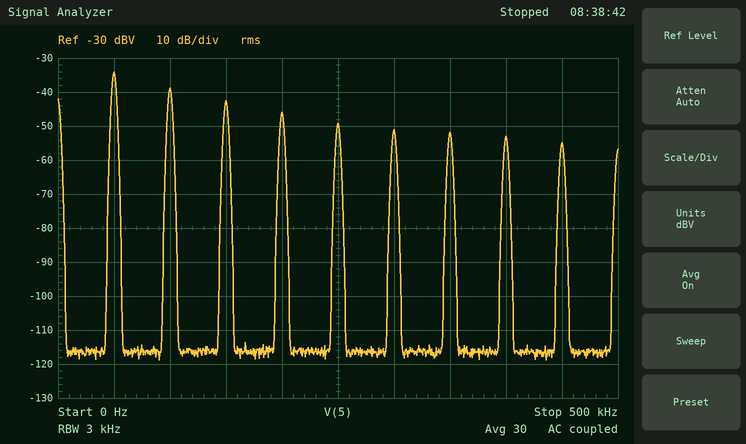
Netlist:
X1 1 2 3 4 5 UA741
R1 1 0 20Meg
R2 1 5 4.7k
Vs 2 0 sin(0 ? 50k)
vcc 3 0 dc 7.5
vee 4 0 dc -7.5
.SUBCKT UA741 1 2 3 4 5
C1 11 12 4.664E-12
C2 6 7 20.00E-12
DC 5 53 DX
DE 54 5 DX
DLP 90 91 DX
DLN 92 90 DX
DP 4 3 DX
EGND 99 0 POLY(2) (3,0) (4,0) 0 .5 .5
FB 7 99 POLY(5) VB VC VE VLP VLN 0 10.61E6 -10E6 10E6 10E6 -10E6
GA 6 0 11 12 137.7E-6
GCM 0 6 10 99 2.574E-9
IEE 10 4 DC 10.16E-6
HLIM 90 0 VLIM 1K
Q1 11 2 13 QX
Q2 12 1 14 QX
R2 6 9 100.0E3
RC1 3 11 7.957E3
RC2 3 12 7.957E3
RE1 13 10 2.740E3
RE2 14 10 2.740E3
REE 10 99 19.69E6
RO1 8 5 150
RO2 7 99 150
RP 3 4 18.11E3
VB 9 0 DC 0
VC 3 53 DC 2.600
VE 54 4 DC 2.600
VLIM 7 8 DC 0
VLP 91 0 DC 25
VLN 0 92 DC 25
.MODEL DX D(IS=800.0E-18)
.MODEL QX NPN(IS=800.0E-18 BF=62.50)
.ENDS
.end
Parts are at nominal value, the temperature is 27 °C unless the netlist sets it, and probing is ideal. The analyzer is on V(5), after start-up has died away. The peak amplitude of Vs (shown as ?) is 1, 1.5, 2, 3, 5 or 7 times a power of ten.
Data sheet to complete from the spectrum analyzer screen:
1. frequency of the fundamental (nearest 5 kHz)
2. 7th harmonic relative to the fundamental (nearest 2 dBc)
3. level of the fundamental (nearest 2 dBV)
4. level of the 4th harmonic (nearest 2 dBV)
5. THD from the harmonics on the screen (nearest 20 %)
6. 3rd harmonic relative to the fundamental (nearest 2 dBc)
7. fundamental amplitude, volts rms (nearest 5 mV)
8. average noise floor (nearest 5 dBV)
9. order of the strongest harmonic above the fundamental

50 kHz
-18 dBc
-34 dBV
-46 dBV
80 %
-8 dBc
20 mV
-115 dBV
2
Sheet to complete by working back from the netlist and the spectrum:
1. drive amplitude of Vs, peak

10 V
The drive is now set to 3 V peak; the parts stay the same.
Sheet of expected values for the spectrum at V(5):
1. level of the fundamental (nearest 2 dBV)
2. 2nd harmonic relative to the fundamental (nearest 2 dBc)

-72 dBV
-50 dBc
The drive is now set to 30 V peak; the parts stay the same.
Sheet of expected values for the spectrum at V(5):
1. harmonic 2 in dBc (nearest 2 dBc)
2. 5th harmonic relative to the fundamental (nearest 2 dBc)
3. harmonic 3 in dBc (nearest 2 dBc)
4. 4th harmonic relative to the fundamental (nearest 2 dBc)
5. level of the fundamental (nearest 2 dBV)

-12 dBc
-24 dBc
-16 dBc
-20 dBc
-28 dBV
